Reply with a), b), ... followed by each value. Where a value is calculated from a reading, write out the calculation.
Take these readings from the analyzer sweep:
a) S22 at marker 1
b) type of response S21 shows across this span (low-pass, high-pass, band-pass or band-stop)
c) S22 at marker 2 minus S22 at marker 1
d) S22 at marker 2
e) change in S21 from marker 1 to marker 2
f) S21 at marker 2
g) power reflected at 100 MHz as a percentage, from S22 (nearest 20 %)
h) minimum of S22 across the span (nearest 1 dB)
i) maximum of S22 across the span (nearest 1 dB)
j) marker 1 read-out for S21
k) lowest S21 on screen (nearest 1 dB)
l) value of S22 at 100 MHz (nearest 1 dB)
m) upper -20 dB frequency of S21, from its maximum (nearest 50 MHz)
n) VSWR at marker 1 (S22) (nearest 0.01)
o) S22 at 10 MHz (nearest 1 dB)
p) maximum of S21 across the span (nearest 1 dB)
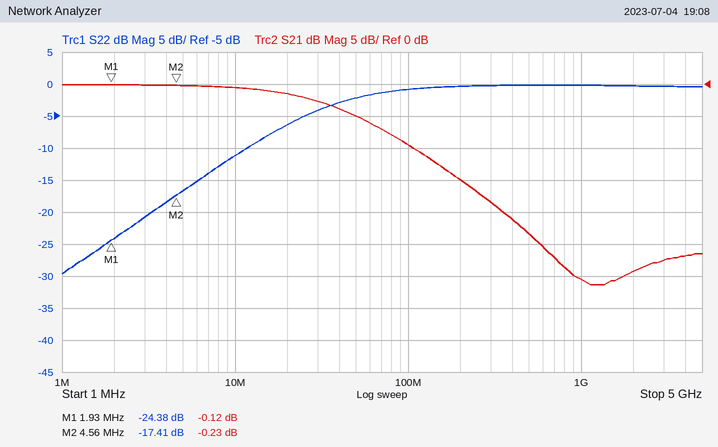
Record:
a) -24.38 dB
b) low-pass
c) -17.41 − (-24.38) = 6.97 dB
d) -17.41 dB
e) -0.23 − (-0.12) = -0.11 dB
f) -0.23 dB
g) 10^(-1/10) ≈ 79.4 %, so 80 % to the nearest 20 %
h) -30 dB
i) 0 dB
j) -0.12 dB
k) -31 dB
l) -1 dB
m) 350 MHz
n) (1 + 0.0604)/(1 − 0.0604) ≈ 1.13
o) -11 dB
p) 0 dB
